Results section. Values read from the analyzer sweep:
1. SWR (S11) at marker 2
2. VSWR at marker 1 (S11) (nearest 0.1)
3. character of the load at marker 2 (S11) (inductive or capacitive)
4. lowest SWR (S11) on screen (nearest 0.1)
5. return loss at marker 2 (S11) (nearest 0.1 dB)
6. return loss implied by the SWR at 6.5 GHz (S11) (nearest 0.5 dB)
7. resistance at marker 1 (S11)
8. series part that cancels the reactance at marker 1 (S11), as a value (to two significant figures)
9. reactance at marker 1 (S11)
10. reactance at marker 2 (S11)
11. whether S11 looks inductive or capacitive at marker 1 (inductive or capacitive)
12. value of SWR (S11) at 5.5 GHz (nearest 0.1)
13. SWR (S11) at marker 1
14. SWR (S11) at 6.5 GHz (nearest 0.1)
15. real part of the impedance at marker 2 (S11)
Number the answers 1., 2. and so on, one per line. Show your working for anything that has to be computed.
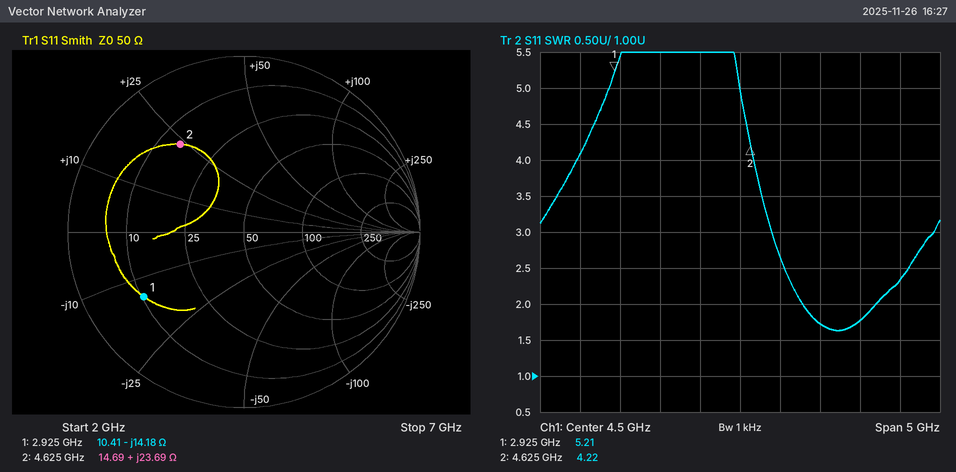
1. 4.22
2. 5.2
3. inductive
4. 1.6
5. 4.2 dB
6. −20 log10((2.3 − 1)/(2.3 + 1)) ≈ 8.09 dB, so 8.0 dB to the nearest 0.5 dB
7. 10.41 Ω
8. L = 14.18 Ω/(2π × 2.925 GHz) ≈ 772 pH, so 770 pH to two significant figures
9. -14.18 Ω
10. +23.69 Ω
11. capacitive
12. 1.7
13. 5.21
14. 2.3
15. 14.69 Ω
